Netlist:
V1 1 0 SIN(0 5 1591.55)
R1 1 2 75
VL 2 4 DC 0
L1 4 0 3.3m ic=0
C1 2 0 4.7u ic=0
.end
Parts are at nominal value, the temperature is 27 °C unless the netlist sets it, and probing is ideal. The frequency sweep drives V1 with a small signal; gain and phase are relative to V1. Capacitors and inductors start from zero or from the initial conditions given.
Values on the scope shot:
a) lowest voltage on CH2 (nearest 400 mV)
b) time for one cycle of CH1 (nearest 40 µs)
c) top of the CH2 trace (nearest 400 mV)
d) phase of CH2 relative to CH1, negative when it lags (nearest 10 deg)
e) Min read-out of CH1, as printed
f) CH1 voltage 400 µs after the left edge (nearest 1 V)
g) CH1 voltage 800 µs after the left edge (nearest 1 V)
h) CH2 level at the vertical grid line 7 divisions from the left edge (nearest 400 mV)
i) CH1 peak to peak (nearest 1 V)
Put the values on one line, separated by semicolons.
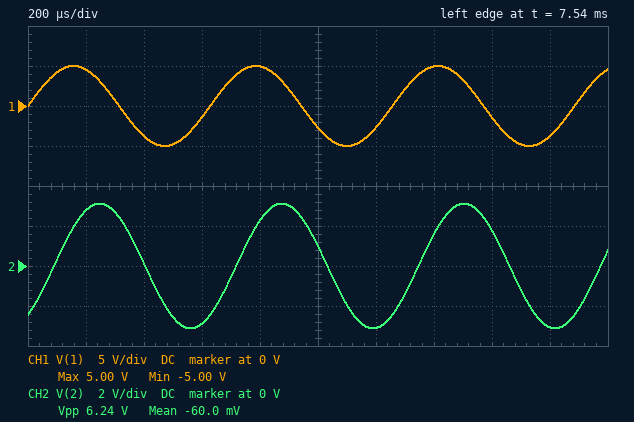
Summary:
-3.2 V; 640 µs; 3.2 V; -50 deg; -5.00 V; -4 V; 5 V; 1.6 V; 10 V
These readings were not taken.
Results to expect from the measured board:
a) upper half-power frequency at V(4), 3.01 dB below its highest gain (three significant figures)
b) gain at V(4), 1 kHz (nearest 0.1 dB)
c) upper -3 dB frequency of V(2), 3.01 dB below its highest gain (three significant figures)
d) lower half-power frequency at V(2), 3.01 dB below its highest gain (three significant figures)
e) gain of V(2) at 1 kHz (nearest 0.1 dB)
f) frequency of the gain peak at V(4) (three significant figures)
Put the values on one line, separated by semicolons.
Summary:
1.52 kHz; -4.7 dB; 1.52 kHz; 1.07 kHz; -4.7 dB; 1.28 kHz
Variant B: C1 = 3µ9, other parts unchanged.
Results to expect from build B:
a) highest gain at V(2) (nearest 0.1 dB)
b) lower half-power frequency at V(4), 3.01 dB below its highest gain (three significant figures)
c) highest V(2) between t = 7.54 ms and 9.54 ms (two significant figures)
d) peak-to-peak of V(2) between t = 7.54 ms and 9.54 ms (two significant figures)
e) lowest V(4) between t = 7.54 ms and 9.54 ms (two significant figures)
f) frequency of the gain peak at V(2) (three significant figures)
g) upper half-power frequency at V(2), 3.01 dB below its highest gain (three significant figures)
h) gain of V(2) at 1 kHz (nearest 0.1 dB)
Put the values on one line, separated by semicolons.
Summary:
0 dB; 1.16 kHz; 4.2 V; 8.4 V; -4.2 V; 1.40 kHz; 1.70 kHz; -6.2 dB
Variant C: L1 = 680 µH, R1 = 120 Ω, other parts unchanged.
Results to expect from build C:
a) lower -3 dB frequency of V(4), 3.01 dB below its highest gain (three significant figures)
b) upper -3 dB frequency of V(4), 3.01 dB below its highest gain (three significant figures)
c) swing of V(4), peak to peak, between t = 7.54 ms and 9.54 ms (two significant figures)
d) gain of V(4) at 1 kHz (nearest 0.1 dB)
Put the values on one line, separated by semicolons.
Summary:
2.68 kHz; 2.96 kHz; 830 mV; -27.8 dB
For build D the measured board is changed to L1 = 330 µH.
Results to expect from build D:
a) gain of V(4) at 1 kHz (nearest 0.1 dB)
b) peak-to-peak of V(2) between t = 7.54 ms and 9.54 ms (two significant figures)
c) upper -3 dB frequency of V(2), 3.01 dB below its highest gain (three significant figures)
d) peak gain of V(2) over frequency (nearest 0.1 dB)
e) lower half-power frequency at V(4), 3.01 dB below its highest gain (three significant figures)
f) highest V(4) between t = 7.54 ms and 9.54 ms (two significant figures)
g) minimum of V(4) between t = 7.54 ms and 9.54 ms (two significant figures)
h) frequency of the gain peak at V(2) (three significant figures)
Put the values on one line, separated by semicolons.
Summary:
-30.6 dB; 520 mV; 4.27 kHz; 0 dB; 3.82 kHz; 260 mV; -260 mV; 4.04 kHz
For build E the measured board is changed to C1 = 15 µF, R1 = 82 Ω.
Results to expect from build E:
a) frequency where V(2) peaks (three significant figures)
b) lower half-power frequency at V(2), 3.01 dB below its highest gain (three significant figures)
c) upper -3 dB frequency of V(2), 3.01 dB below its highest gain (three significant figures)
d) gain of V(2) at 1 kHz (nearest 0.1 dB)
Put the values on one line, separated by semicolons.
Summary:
715 Hz; 654 Hz; 783 Hz; -11.8 dB
